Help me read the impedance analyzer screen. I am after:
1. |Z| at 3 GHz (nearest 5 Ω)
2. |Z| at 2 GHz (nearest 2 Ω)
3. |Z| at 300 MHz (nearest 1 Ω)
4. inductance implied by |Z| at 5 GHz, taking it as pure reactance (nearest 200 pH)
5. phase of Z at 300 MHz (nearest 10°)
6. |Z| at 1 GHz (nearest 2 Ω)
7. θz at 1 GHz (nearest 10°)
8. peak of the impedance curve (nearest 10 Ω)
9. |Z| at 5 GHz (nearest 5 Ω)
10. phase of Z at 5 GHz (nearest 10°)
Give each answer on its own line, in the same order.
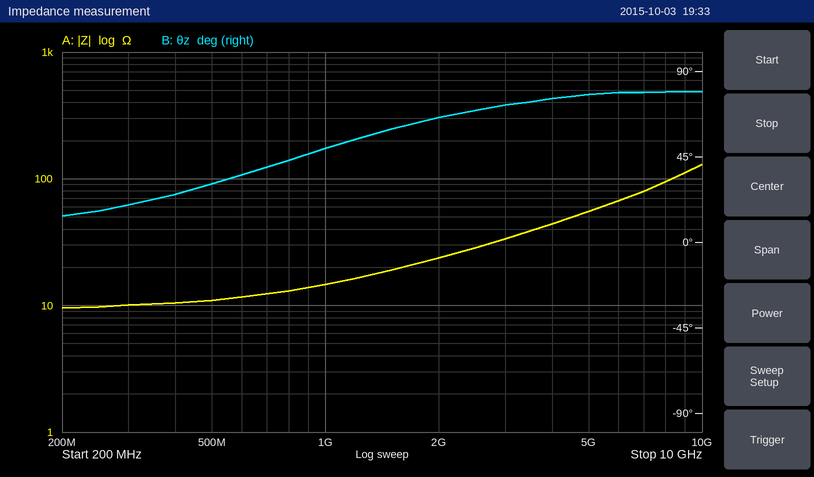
35 Ω
24 Ω
10 Ω
1.8 nH
20°
14 Ω
50°
130 Ω
55 Ω
80°
